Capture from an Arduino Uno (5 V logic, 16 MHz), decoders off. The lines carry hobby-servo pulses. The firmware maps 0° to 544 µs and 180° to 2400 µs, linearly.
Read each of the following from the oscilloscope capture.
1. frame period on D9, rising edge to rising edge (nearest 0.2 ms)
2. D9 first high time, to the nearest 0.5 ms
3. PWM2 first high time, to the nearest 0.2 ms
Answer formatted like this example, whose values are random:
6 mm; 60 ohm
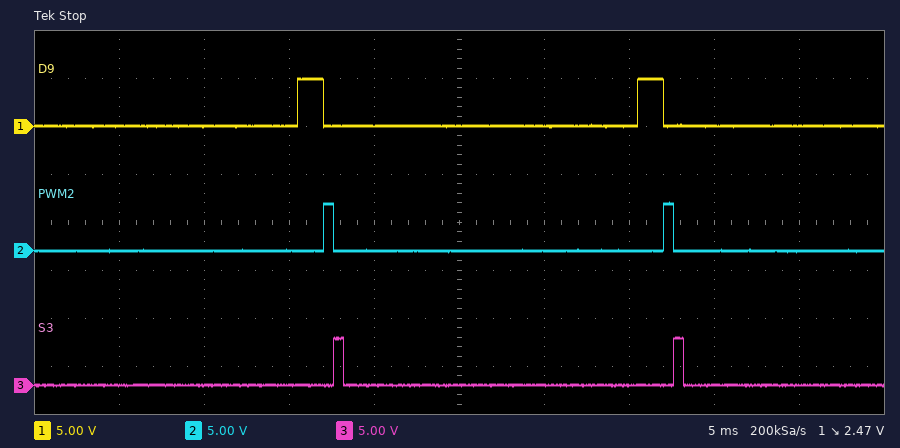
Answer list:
20.0 ms; 1.5 ms; 0.6 ms
